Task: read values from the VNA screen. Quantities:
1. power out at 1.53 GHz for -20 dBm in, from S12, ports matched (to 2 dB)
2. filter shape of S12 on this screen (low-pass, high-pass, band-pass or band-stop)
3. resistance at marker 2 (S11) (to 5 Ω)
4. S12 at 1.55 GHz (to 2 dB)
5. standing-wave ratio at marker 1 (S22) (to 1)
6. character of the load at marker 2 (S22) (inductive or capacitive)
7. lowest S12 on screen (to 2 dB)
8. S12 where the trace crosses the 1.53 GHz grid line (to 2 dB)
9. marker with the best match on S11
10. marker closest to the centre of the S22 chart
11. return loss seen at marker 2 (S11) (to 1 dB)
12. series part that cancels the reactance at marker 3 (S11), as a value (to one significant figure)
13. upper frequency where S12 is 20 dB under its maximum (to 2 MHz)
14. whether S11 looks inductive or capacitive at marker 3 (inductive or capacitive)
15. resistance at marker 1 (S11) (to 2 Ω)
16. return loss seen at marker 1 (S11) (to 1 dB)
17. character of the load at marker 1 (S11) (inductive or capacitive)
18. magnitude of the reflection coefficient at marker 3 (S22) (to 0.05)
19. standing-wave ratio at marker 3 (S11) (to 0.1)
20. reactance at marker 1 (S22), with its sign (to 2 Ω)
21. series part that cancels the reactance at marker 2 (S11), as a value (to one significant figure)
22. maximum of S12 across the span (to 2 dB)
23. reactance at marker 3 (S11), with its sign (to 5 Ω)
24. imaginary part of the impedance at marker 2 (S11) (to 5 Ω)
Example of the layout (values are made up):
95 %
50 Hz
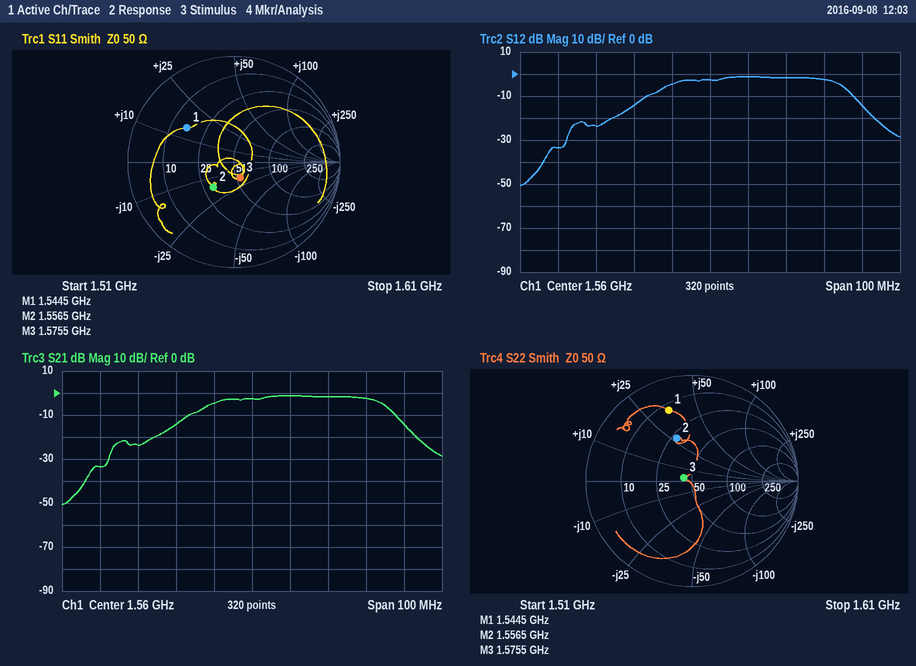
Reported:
-44 dBm
band-pass
30 Ω
-4 dB
6
inductive
-50 dB
-24 dB
marker 3
marker 3
10 dB
2 nH
1.604 GHz
capacitive
16 Ω
5 dB
inductive
0.10
1.4
+34 Ω
2 nH
-2 dB
-15 Ω
-15 Ω
